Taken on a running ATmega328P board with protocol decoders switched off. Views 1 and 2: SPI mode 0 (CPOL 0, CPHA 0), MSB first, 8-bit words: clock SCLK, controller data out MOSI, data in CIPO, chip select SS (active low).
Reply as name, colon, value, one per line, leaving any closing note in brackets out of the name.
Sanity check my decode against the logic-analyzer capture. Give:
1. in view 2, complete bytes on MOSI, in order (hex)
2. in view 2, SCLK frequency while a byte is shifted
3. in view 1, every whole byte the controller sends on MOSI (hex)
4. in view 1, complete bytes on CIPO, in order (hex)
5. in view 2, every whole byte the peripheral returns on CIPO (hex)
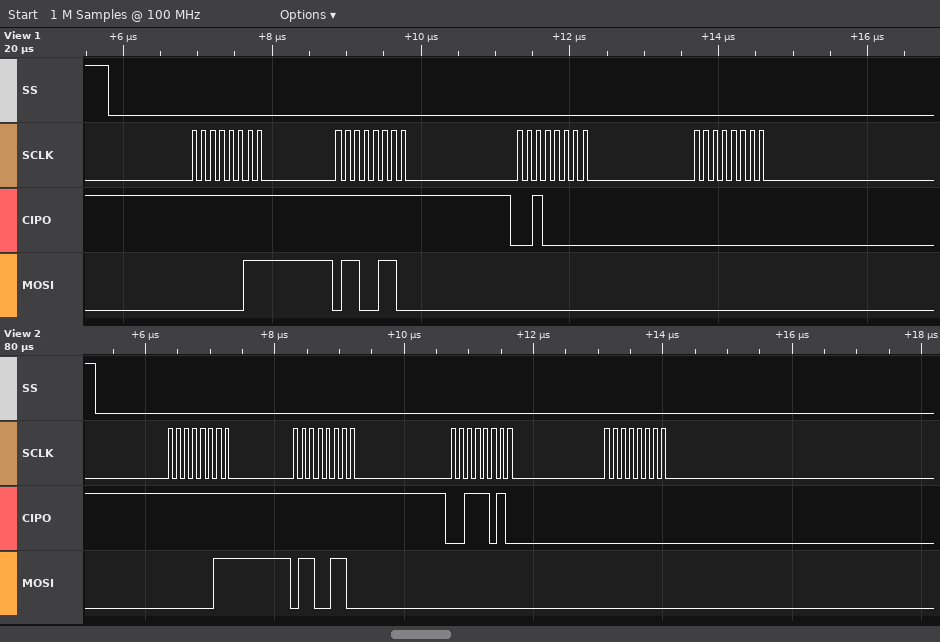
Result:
in view 2, complete bytes on MOSI, in order: 03 66 00 00
in view 2, SCLK frequency while a byte is shifted: 8 MHz
in view 1, every whole byte the controller sends on MOSI: 03 66 00 00
in view 1, complete bytes on CIPO, in order: FF FF 20 00
in view 2, every whole byte the peripheral returns on CIPO: FF FF 3A 00
